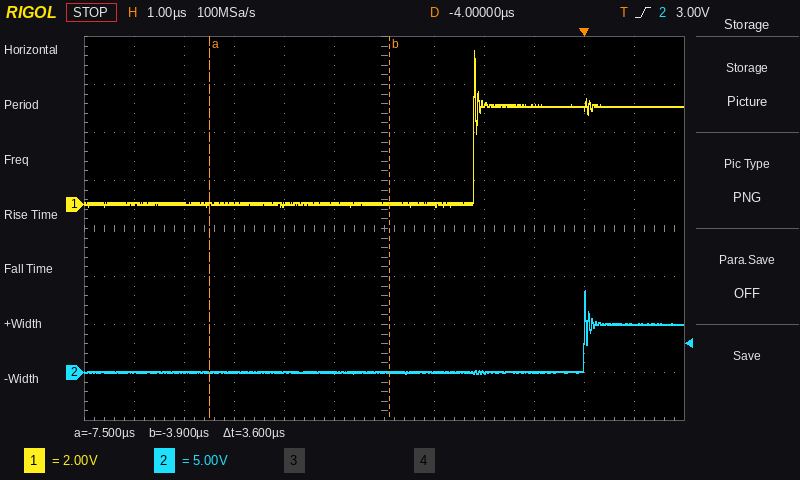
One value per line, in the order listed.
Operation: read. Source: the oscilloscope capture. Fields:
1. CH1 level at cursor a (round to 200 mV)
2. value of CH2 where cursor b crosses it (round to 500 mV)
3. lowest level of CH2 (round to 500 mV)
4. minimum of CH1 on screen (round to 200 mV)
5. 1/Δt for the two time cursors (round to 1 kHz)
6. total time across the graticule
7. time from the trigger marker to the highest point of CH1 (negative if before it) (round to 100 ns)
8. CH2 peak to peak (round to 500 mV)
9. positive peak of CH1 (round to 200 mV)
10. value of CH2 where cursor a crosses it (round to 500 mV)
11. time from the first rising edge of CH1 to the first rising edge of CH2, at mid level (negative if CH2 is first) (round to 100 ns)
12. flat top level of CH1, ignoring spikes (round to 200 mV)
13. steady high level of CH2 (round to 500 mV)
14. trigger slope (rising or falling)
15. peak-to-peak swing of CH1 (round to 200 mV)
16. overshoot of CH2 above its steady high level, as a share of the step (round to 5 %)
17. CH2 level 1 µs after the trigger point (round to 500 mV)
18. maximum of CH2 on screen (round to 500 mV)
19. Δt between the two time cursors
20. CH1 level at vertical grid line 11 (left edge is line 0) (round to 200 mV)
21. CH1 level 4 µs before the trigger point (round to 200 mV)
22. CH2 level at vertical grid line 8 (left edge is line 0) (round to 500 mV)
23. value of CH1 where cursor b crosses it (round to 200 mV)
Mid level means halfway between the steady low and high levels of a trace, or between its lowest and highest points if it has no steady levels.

0.0 V
0.0 V
0.0 V
0.0 V
278 kHz
12 µs
-2.2 µs
8.5 V
6.4 V
0.0 V
+2.2 µs
4.0 V
5.0 V
rising
6.4 V
70 %
5.0 V
8.5 V
3.6 µs
4.0 V
0.0 V
0.0 V
0.0 V
